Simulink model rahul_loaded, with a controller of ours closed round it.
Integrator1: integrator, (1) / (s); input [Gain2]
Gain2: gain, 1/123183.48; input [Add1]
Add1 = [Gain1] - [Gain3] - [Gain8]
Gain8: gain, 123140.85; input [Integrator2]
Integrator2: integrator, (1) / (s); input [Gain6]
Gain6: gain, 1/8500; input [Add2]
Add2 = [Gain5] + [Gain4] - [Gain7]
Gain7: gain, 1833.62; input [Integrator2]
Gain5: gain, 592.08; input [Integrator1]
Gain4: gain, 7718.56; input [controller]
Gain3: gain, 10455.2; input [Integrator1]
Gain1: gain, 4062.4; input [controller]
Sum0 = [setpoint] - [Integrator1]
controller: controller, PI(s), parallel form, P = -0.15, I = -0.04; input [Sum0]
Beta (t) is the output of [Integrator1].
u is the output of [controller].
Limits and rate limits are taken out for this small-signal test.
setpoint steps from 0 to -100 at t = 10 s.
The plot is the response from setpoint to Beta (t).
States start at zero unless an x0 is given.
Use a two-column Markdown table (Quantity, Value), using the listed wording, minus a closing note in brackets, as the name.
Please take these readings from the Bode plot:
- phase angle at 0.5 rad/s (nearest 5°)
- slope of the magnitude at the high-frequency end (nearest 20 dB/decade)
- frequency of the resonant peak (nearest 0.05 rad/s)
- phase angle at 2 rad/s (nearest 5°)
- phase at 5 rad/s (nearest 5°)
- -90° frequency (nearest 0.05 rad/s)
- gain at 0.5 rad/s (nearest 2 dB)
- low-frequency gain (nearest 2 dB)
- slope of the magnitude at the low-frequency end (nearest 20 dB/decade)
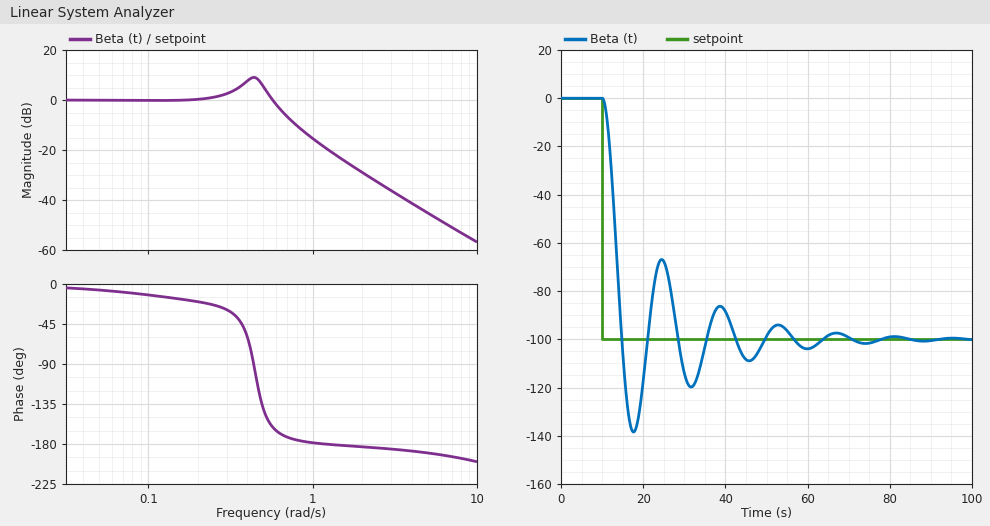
| Quantity | Value |
|---|---|
| phase angle at 0.5 rad/s | -140° |
| slope of the magnitude at the high-frequency end | -40 dB/decade |
| frequency of the resonant peak | 0.45 rad/s |
| phase angle at 2 rad/s | -185° |
| phase at 5 rad/s | -190° |
| -90° frequency | 0.45 rad/s |
| gain at 0.5 rad/s | 6 dB |
| low-frequency gain | 0 dB |
| slope of the magnitude at the low-frequency end | 0 dB/decade |
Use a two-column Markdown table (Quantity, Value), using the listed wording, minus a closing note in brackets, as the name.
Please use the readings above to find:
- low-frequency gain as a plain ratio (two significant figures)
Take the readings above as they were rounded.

| Quantity | Value |
|---|---|
| low-frequency gain as a plain ratio | 1.0 |
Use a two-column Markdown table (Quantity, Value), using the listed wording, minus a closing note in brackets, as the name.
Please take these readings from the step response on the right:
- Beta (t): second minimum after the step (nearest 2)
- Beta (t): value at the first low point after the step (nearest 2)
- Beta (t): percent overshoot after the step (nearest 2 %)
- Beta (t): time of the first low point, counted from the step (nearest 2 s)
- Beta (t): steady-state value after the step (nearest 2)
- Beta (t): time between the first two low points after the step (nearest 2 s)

| Quantity | Value |
|---|---|
| Beta (t): second minimum after the step | -120 |
| Beta (t): value at the first low point after the step | -138 |
| Beta (t): percent overshoot after the step | 38 % |
| Beta (t): time of the first low point, counted from the step | 8 s |
| Beta (t): steady-state value after the step | -100 |
| Beta (t): time between the first two low points after the step | 14 s |
